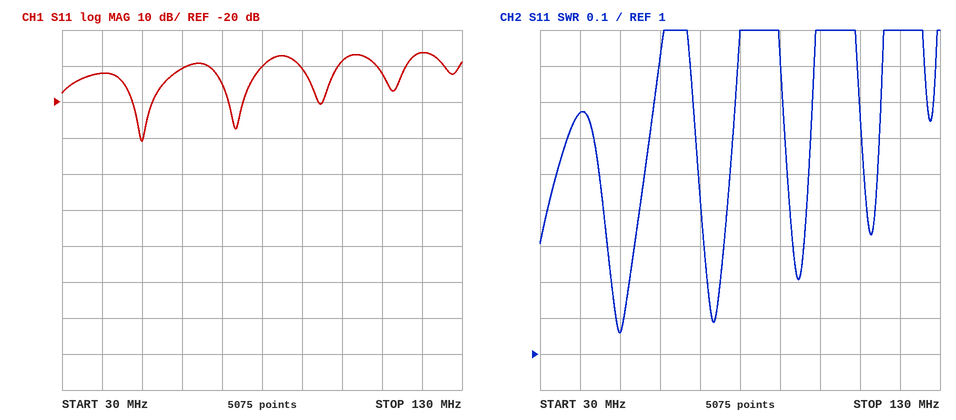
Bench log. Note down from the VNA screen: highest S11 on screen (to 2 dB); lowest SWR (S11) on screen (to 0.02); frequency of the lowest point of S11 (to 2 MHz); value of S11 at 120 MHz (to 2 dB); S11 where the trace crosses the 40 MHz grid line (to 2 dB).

-6 dB
1.06
50 MHz
-6 dB
-12 dB
